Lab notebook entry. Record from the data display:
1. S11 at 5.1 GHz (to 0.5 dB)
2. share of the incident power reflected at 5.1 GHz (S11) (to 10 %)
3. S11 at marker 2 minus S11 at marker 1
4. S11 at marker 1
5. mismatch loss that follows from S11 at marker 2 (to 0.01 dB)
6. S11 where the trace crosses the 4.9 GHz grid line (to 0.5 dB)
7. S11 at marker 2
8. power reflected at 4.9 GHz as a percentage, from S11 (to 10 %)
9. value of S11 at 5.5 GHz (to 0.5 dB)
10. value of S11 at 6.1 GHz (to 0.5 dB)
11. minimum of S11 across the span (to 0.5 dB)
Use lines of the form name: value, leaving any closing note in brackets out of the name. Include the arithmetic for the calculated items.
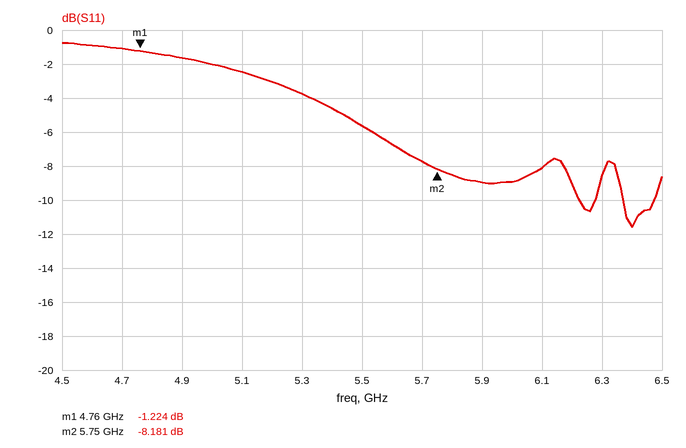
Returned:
S11 at 5.1 GHz: -2.5 dB
share of the incident power reflected at 5.1 GHz (S11): 10^(-2.5/10) ≈ 56.2 %, so 60 % to the nearest 10 %
S11 at marker 2 minus S11 at marker 1: -8.181 − (-1.224) = -6.957 dB
S11 at marker 1: -1.224 dB
mismatch loss that follows from S11 at marker 2: −10 log10(1 − 10^(-8.181/10)) ≈ 0.72 dB
S11 where the trace crosses the 4.9 GHz grid line: -1.5 dB
S11 at marker 2: -8.181 dB
power reflected at 4.9 GHz as a percentage, from S11: 10^(-1.5/10) ≈ 70.8 %, so 70 % to the nearest 10 %
value of S11 at 5.5 GHz: -5.5 dB
value of S11 at 6.1 GHz: -8.0 dB
minimum of S11 across the span: -11.5 dB
